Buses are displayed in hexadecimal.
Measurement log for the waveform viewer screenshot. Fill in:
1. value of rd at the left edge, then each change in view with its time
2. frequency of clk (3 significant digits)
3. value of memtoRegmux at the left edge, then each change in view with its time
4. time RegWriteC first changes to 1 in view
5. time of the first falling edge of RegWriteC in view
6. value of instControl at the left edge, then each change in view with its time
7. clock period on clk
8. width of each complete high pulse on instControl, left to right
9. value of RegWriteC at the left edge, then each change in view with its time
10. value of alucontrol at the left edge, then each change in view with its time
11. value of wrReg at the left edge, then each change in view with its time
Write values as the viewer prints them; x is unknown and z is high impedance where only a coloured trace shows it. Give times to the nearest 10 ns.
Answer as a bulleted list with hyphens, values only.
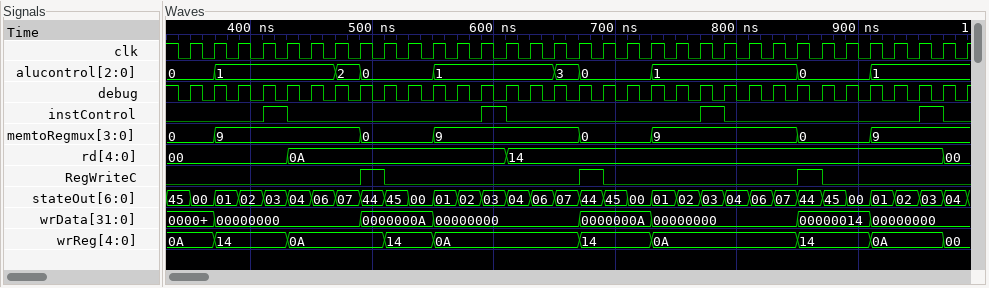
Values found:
- 00, 0A at 430 ns, 14 at 610 ns, 00 at 970 ns
- 50.0 MHz
- 0, 9 at 370 ns, 0 at 490 ns, 9 at 550 ns, 0 at 670 ns, 9 at 730 ns, 0 at 850 ns, 9 at 910 ns
- 490 ns
- 510 ns
- 0, 1 at 410 ns, 0 at 430 ns, 1 at 590 ns, 0 at 610 ns, 1 at 770 ns, 0 at 790 ns, 1 at 950 ns, 0 at 970 ns
- 20 ns
- 20 ns, 20 ns, 20 ns, 20 ns
- 0, 1 at 490 ns, 0 at 510 ns, 1 at 670 ns, 0 at 690 ns, 1 at 850 ns, 0 at 870 ns
- 0, 1 at 370 ns, 2 at 470 ns, 0 at 490 ns, 1 at 550 ns, 3 at 650 ns, 0 at 670 ns, 1 at 730 ns, 0 at 850 ns, 1 at 910 ns
- 0A, 14 at 370 ns, 0A at 430 ns, 14 at 510 ns, 0A at 550 ns, 14 at 670 ns, 0A at 730 ns, 14 at 850 ns, 0A at 910 ns, 00 at 970 ns
